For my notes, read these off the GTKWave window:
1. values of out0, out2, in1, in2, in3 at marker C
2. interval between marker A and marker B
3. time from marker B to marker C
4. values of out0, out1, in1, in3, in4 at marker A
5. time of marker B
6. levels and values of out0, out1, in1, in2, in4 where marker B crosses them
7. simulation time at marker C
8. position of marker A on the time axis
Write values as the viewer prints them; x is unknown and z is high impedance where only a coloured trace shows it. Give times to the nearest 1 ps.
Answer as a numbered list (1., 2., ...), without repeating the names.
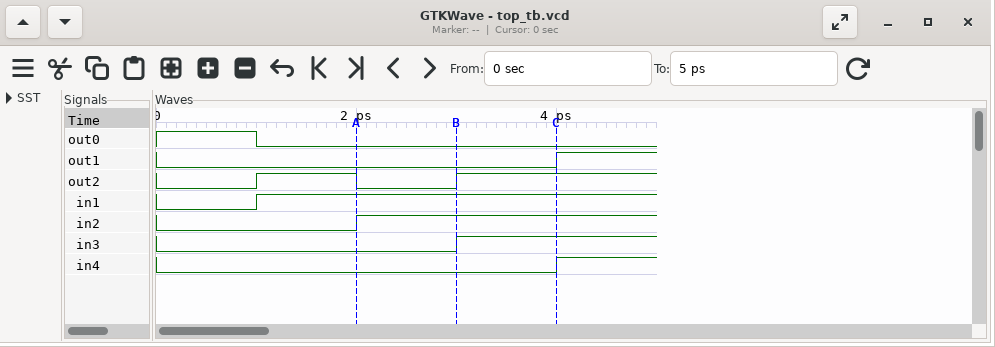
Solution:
1. out0=0, out2=1, in1=1, in2=1, in3=1
2. 1 ps
3. 1 ps
4. out0=0, out1=0, in1=1, in3=0, in4=0
5. 3 ps
6. out0=0, out1=0, in1=1, in2=1, in4=0
7. 4 ps
8. 2 ps
